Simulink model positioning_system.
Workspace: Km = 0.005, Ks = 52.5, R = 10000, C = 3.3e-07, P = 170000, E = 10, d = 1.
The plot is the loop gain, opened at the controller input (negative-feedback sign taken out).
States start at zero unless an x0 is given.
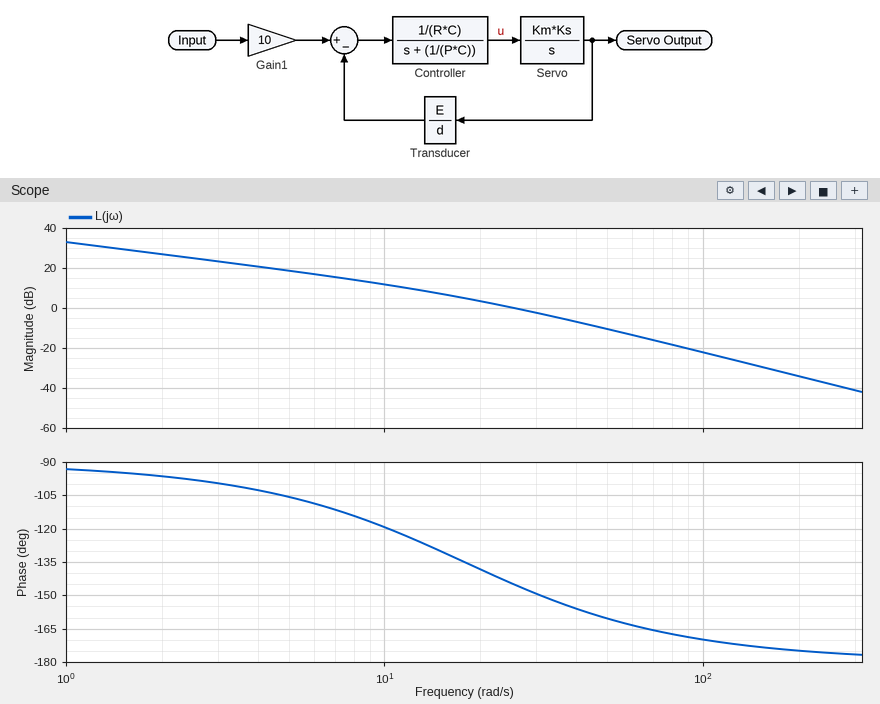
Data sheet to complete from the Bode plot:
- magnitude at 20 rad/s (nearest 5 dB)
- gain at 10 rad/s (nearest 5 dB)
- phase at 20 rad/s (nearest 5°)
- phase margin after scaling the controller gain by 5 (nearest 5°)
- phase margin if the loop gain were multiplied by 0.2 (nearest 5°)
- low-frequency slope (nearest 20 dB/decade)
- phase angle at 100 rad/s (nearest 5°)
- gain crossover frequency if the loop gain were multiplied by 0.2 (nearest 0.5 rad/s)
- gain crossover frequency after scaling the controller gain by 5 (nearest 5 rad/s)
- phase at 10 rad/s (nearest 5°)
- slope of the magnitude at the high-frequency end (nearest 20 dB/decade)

5 dB
10 dB
-140°
15°
65°
-20 dB/decade
-170°
8.0 rad/s
60 rad/s
-120°
-40 dB/decade
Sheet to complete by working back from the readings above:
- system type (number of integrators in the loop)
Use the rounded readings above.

1
